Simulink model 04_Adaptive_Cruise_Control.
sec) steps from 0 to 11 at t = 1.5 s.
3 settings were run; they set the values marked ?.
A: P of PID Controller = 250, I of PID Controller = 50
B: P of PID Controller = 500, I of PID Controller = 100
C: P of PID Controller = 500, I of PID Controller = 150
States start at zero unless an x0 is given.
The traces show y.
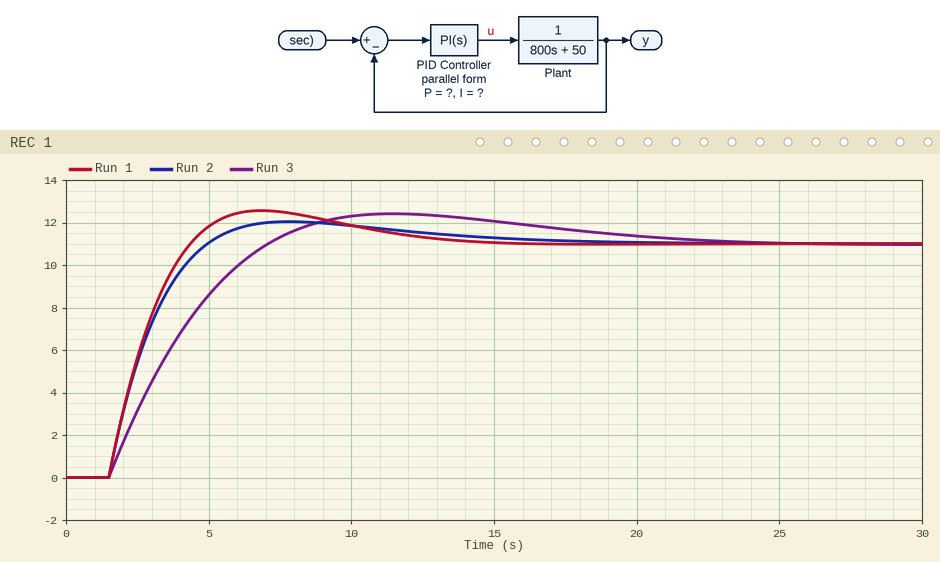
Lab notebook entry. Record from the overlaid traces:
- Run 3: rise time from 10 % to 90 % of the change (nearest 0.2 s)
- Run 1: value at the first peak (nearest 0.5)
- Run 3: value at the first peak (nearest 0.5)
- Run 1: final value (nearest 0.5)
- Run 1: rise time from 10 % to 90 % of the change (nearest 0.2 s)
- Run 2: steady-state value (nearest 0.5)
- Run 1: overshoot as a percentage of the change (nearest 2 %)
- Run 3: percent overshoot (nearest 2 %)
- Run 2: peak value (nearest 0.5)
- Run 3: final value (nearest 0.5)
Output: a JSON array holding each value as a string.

["4.2 s", "12.5", "12.5", "11.0", "2.2 s", "11.0", "14 %", "12 %", "12.0", "11.0"]
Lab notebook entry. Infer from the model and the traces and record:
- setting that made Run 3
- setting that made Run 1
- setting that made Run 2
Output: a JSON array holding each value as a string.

["A", "C", "B"]
